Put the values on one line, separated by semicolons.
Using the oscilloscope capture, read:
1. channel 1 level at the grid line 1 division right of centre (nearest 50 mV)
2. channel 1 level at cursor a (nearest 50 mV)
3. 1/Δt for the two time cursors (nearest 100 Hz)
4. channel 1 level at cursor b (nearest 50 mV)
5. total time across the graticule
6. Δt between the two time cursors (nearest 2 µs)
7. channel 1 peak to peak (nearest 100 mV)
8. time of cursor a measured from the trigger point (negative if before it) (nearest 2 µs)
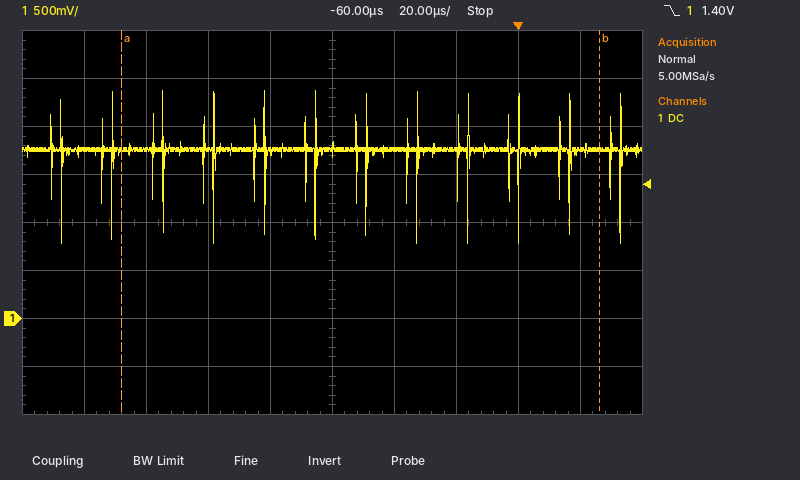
1.75 V; 1.75 V; 6.5 kHz; 1.75 V; 200 µs; 154 µs; 1.60 V; -128 µs
